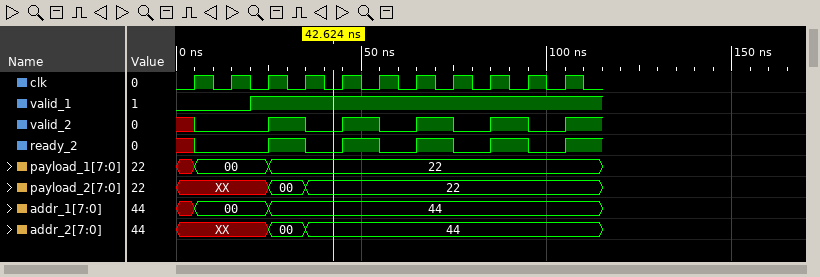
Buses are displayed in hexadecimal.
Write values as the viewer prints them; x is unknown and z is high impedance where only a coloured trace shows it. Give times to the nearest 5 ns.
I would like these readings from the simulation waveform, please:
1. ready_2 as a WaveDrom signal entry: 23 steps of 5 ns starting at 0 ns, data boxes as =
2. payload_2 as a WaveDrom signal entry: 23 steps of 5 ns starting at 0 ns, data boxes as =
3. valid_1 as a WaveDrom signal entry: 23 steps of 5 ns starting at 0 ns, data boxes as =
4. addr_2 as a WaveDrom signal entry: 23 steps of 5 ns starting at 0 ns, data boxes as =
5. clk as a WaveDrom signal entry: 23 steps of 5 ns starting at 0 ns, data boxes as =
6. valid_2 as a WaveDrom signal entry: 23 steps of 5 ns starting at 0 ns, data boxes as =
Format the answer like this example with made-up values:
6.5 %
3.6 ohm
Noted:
{name: 'ready_2', wave: 'x0...1.0.1.0.1.0.1.0.1.'}
{name: 'payload_2', wave: 'x....=.=...............', data: '00 22'}
{name: 'valid_1', wave: '0...1..................'}
{name: 'addr_2', wave: 'x....=.=...............', data: '00 44'}
{name: 'clk', wave: '01010101010101010101010'}
{name: 'valid_2', wave: 'x0...1.0.1.0.1.0.1.0.1.'}
